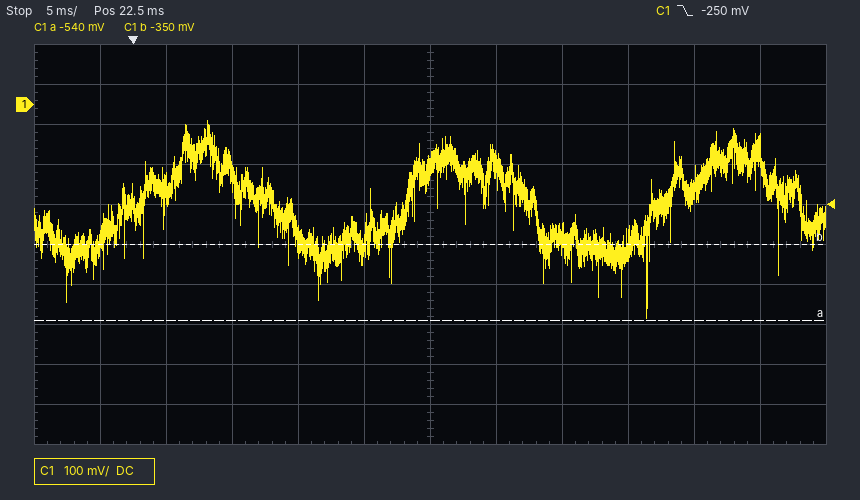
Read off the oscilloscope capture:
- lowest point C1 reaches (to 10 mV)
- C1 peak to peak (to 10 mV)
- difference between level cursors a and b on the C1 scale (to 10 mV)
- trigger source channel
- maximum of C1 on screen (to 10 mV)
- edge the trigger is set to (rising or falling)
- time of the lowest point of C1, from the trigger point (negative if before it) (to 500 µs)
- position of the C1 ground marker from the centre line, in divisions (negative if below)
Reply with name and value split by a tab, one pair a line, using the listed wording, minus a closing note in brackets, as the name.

lowest point C1 reaches	-540 mV
C1 peak to peak	500 mV
difference between level cursors a and b on the C1 scale	190 mV
trigger source channel	C1
maximum of C1 on screen	-40 mV
edge the trigger is set to	falling
time of the lowest point of C1, from the trigger point (negative if before it)	+39.0 ms
position of the C1 ground marker from the centre line, in divisions	+3.5 div
